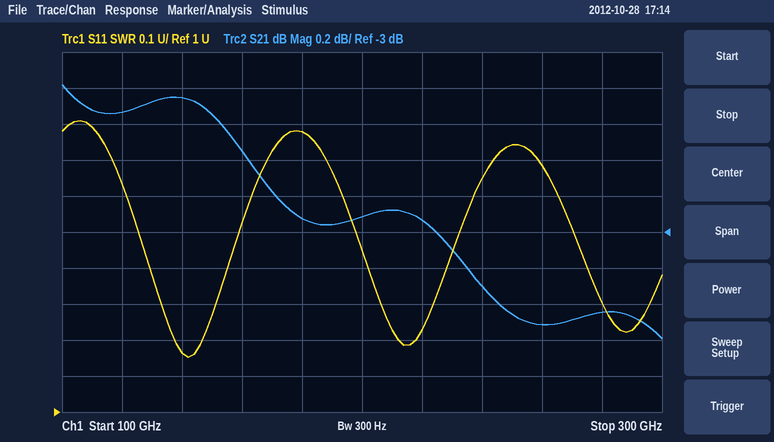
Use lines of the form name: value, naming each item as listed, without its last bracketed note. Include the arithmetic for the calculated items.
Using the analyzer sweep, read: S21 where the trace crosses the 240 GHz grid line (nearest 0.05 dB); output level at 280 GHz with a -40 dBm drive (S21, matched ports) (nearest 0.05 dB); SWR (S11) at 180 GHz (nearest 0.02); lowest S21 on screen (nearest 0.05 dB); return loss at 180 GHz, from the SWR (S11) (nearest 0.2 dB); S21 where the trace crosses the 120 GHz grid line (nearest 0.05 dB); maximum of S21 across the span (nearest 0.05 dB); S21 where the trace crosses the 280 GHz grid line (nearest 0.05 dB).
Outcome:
S21 where the trace crosses the 240 GHz grid line: -3.30 dB
output level at 280 GHz with a -40 dBm drive (S21, matched ports): -40 dBm + (-3.45 dB) = -43.45 dBm
SWR (S11) at 180 GHz: 1.78
lowest S21 on screen: -3.60 dB
return loss at 180 GHz, from the SWR (S11): −20 log10((1.78 − 1)/(1.78 + 1)) ≈ 11.0 dB
S21 where the trace crosses the 120 GHz grid line: -2.35 dB
maximum of S21 across the span: -2.20 dB
S21 where the trace crosses the 280 GHz grid line: -3.45 dB
